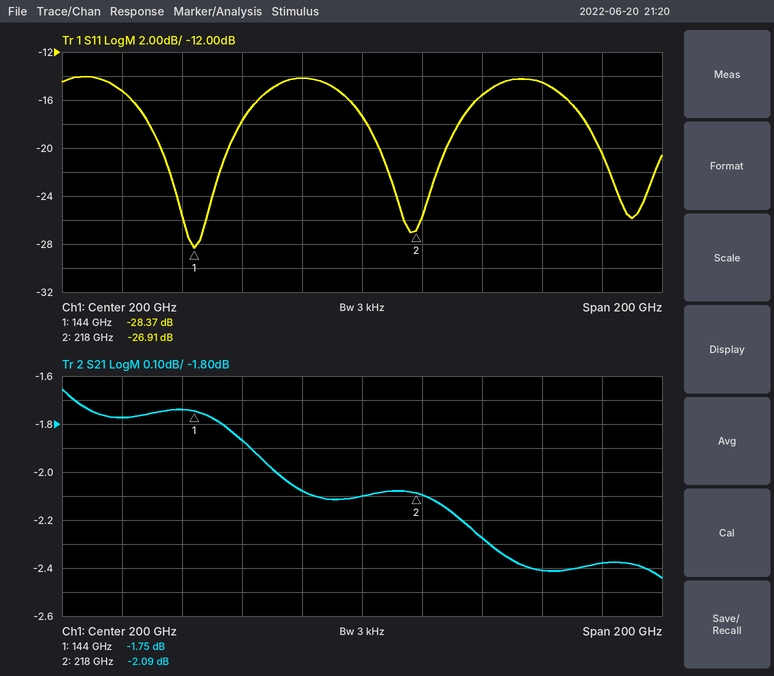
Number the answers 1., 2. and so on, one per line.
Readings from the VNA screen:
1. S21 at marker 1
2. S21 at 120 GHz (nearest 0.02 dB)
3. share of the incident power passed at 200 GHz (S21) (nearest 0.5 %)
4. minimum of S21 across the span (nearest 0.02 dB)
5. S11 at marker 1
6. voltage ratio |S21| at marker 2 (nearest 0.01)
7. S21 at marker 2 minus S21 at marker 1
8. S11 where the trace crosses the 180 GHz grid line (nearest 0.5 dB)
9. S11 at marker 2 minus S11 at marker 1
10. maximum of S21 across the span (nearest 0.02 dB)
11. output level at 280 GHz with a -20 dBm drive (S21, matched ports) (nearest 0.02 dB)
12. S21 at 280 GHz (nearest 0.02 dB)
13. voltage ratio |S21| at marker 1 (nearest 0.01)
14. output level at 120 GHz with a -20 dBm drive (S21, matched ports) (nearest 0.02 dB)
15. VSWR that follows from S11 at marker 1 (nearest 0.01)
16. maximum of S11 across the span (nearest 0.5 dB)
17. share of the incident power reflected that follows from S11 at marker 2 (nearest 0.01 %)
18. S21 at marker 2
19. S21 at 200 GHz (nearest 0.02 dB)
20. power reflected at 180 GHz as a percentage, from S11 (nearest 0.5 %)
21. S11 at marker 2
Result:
1. -1.75 dB
2. -1.78 dB
3. 61.5 %
4. -2.44 dB
5. -28.37 dB
6. 0.79
7. -0.34 dB
8. -14.0 dB
9. 1.46 dB
10. -1.66 dB
11. -22.38 dBm
12. -2.38 dB
13. 0.82
14. -21.78 dBm
15. 1.08
16. -14.0 dB
17. 0.20 %
18. -2.09 dB
19. -2.10 dB
20. 4.0 %
21. -26.91 dB
